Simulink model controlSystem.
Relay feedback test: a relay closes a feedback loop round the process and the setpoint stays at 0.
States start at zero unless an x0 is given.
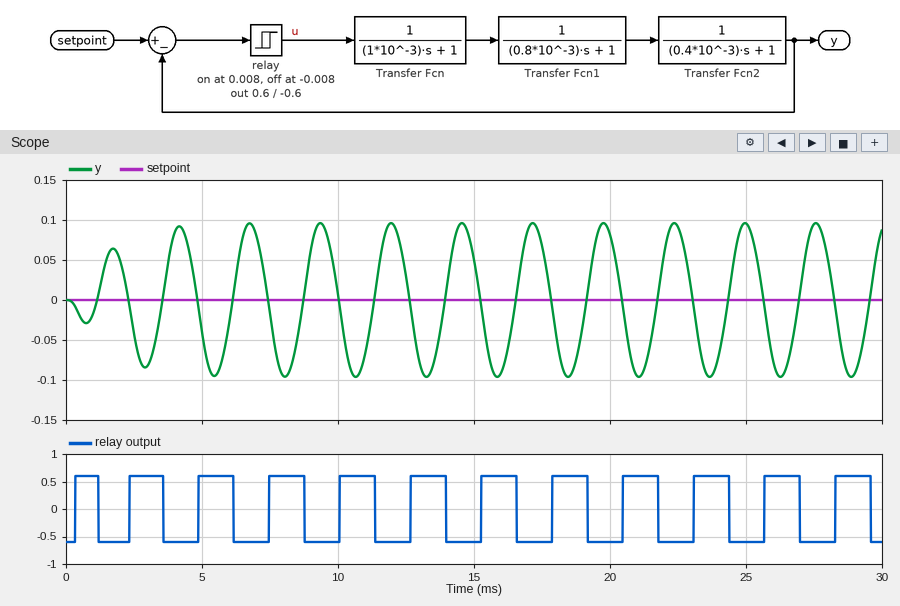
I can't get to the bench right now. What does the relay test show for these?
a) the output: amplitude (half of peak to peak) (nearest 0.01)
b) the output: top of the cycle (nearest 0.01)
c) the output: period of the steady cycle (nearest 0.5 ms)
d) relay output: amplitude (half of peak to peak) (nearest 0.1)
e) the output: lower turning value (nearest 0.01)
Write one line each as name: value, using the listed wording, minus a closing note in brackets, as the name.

the output: amplitude (half of peak to peak): 0.10
the output: top of the cycle: 0.10
the output: period of the steady cycle: 2.5 ms
relay output: amplitude (half of peak to peak): 0.6
the output: lower turning value: -0.10
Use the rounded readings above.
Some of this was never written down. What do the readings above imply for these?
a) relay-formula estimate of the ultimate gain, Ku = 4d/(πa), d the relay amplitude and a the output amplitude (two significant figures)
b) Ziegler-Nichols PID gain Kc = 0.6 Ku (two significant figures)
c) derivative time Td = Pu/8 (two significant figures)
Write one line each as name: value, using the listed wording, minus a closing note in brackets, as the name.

relay-formula estimate of the ultimate gain, Ku = 4d/(πa), d the relay amplitude and a the output amplitude: 7.6
Ziegler-Nichols PID gain Kc = 0.6 Ku: 4.6
derivative time Td = Pu/8: 0.31 ms
